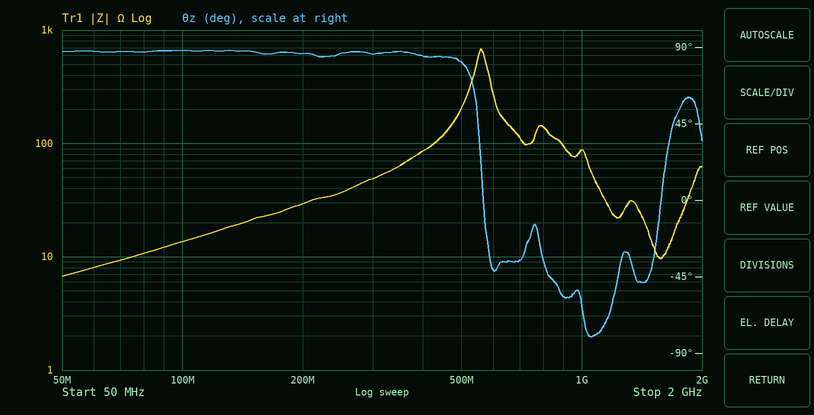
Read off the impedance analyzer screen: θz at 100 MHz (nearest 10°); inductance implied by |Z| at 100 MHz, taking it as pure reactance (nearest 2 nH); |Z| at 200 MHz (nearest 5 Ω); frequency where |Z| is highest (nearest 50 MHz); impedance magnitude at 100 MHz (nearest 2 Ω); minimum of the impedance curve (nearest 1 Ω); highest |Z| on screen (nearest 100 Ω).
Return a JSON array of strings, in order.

["90°", "22 nH", "30 Ω", "550 MHz", "14 Ω", "7 Ω", "700 Ω"]
